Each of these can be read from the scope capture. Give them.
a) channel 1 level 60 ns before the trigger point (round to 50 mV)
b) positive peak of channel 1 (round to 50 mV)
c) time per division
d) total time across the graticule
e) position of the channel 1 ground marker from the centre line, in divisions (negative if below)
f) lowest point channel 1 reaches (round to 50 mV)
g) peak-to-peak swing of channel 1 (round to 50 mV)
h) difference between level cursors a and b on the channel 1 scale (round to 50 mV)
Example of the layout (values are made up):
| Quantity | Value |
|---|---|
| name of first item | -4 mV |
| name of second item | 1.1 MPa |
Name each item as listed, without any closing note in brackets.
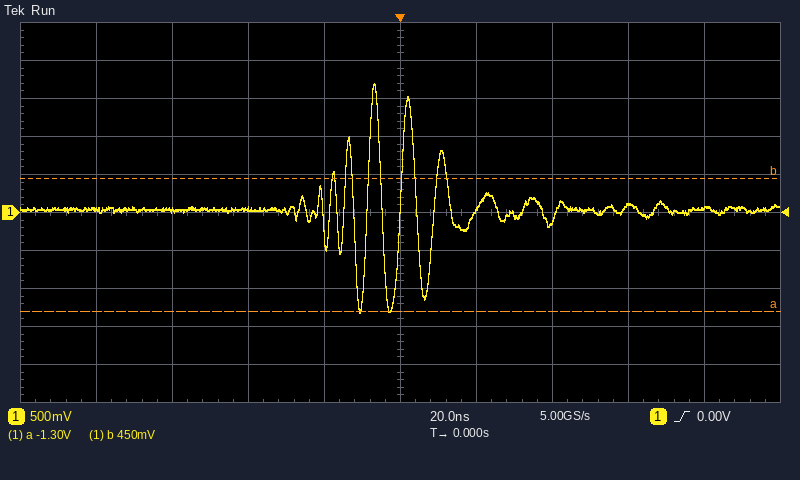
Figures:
| Quantity | Value |
|---|---|
| channel 1 level 60 ns before the trigger point | 50 mV |
| positive peak of channel 1 | 1.70 V |
| time per division | 20 ns |
| total time across the graticule | 200 ns |
| position of the channel 1 ground marker from the centre line, in divisions | 0.0 div |
| lowest point channel 1 reaches | -1.30 V |
| peak-to-peak swing of channel 1 | 3.00 V |
| difference between level cursors a and b on the channel 1 scale | 1.75 V |
